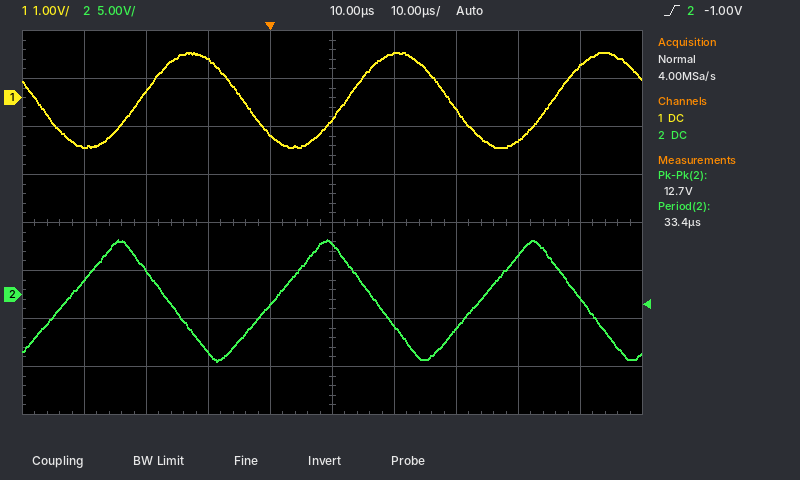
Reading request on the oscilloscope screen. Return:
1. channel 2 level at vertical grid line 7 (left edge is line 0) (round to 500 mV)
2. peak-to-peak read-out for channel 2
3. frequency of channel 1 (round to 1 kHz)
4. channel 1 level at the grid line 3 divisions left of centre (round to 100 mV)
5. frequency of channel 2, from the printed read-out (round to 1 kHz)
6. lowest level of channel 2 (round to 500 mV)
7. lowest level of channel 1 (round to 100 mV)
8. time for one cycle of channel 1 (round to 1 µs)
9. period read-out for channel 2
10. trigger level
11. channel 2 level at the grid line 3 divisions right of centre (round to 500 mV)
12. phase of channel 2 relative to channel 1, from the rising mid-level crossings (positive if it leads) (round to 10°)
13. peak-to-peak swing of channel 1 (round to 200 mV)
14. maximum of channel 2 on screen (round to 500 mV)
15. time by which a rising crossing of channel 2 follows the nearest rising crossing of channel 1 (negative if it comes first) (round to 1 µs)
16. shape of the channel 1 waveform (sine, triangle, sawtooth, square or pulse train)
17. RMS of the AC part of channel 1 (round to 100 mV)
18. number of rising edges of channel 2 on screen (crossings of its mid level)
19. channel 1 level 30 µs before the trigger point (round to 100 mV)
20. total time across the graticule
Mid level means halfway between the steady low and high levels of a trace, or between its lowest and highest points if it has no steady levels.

-3.5 V
12.7 V
30 kHz
100 mV
30 kHz
-7.0 V
-1.0 V
33 µs
33.4 µs
-1.00 V
4.0 V
+130°
2.0 V
5.5 V
-12 µs
sine
700 mV
3
-1.0 V
100 µs
